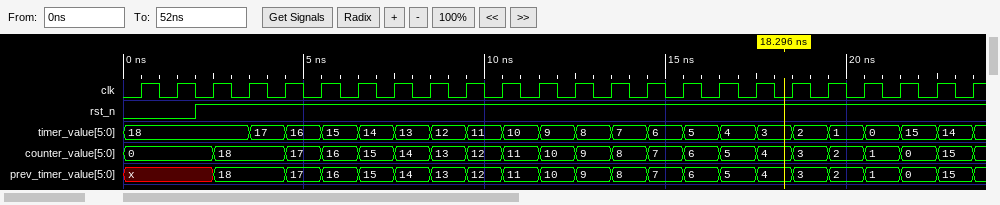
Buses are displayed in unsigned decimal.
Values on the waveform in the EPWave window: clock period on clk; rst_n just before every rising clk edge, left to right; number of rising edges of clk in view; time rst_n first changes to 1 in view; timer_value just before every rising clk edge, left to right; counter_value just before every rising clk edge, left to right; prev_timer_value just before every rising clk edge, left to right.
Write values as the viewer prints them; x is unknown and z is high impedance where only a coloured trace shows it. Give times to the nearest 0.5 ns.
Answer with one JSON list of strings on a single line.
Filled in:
["1 ns", "0 0 1 1 1 1 1 1 1 1 1 1 1 1 1 1 1 1 1 1 1 1 1 1", "24", "2 ns", "18, 18, 18, 18, 17, 16, 15, 14, 13, 12, 11, 10, 9, 8, 7, 6, 5, 4, 3, 2, 1, 0, 15, 14", "0, 0, 0, 18, 18, 17, 16, 15, 14, 13, 12, 11, 10, 9, 8, 7, 6, 5, 4, 3, 2, 1, 0, 15", "x, x, x, 18, 18, 17, 16, 15, 14, 13, 12, 11, 10, 9, 8, 7, 6, 5, 4, 3, 2, 1, 0, 15"]
